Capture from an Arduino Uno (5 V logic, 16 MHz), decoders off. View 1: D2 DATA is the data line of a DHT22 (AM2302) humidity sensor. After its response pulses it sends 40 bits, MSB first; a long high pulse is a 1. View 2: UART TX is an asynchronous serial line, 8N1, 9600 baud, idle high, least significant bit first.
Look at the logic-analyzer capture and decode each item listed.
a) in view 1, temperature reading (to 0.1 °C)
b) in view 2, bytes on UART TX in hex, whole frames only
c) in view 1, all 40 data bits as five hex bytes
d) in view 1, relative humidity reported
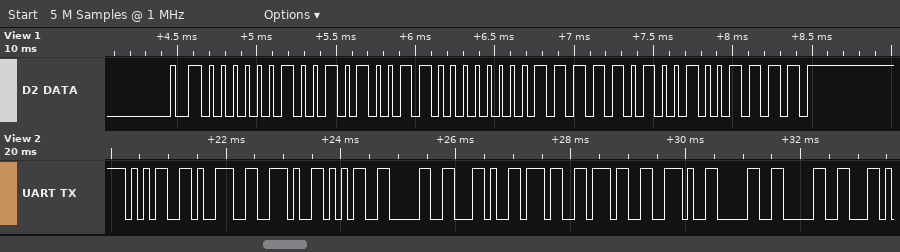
25.0 °C
35 39 2E 35 30 2C 37 37 2E 30 30
02 53 00 FA 4F
59.5 %
